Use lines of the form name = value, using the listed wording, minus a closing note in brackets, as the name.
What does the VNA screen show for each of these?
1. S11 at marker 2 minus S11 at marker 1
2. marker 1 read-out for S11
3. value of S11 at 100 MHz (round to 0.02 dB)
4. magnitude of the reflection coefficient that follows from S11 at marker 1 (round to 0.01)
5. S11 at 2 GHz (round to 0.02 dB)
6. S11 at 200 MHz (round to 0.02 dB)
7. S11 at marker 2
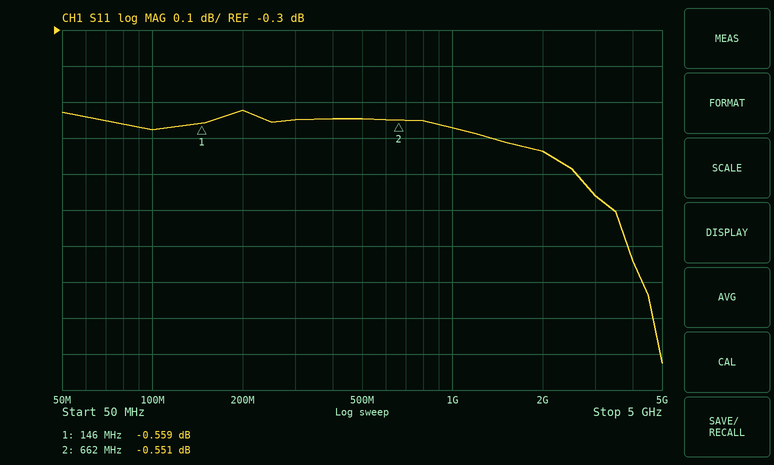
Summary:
S11 at marker 2 minus S11 at marker 1 = 0.008 dB
marker 1 read-out for S11 = -0.559 dB
value of S11 at 100 MHz = -0.58 dB
magnitude of the reflection coefficient that follows from S11 at marker 1 = 0.94
S11 at 2 GHz = -0.64 dB
S11 at 200 MHz = -0.52 dB
S11 at marker 2 = -0.551 dB
